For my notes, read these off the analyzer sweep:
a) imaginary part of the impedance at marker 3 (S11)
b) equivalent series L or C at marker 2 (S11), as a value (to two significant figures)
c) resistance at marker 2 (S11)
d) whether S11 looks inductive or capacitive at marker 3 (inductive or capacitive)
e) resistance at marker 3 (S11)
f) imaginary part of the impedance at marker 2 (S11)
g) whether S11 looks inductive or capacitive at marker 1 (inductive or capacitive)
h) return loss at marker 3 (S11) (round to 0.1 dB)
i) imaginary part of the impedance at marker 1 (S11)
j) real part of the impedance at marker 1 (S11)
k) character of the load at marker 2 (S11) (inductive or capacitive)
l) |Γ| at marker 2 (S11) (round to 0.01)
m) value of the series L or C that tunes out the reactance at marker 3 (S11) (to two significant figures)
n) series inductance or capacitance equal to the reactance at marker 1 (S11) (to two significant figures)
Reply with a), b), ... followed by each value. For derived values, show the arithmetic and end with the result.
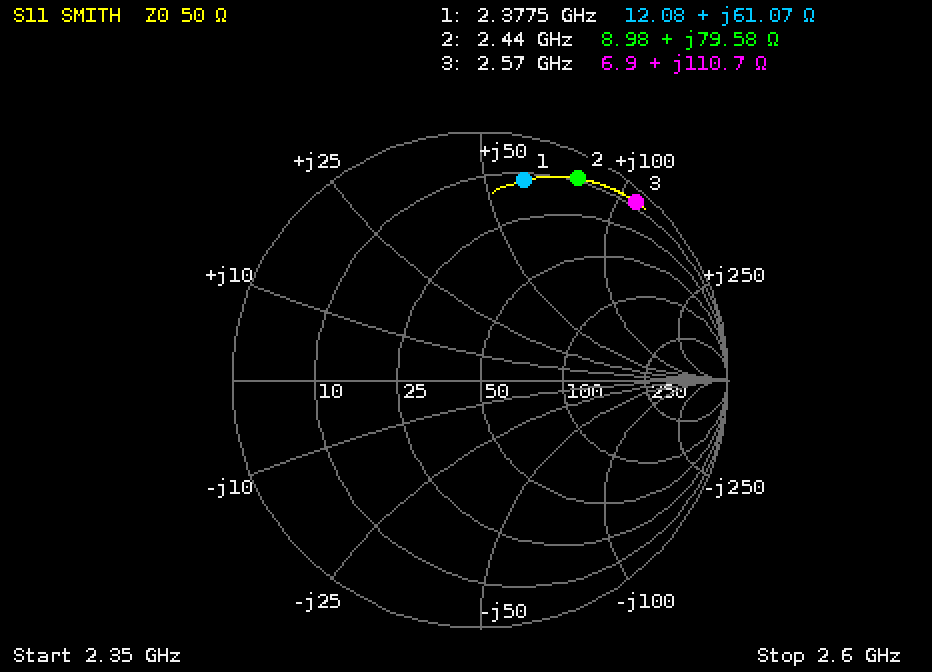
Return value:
a) +110.7 Ω
b) L = 79.58 Ω/(2π × 2.44 GHz) ≈ 5.2 nH
c) 8.98 Ω
d) inductive
e) 6.9 Ω
f) +79.58 Ω
g) inductive
h) 0.4 dB
i) +61.07 Ω
j) 12.08 Ω
k) inductive
l) 0.90
m) C = 1/(2π × 2.57 GHz × 110.7 Ω) ≈ 559 fF, so 560 fF to two significant figures
n) L = 61.07 Ω/(2π × 2.3775 GHz) ≈ 4.1 nH
